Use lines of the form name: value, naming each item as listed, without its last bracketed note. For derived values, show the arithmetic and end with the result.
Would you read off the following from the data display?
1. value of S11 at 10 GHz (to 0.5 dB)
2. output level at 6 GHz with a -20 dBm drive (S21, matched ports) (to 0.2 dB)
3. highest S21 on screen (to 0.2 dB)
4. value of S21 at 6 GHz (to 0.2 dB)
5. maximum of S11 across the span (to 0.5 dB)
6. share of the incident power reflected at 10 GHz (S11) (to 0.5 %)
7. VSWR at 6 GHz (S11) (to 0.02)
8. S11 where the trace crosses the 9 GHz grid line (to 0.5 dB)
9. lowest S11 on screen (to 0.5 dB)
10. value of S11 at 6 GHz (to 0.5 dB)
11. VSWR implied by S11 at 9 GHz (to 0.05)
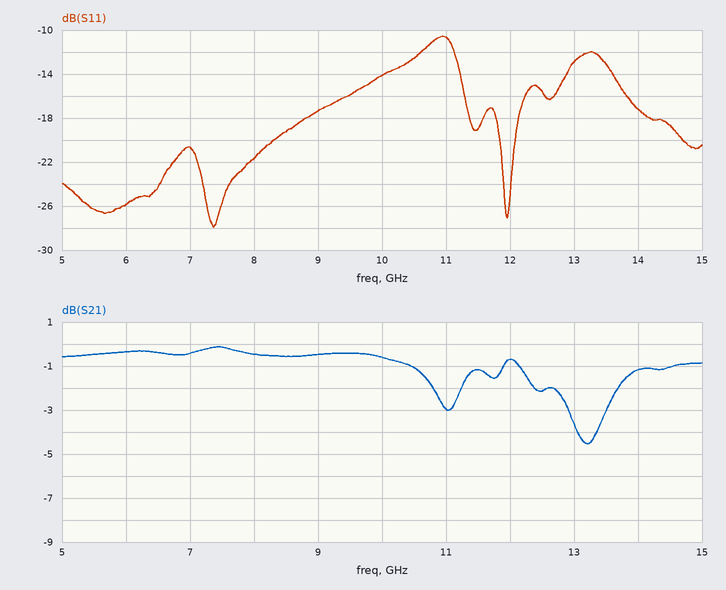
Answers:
value of S11 at 10 GHz: -14.0 dB
output level at 6 GHz with a -20 dBm drive (S21, matched ports): -20 dBm + (-0.4 dB) = -20.4 dBm
highest S21 on screen: -0.2 dB
value of S21 at 6 GHz: -0.4 dB
maximum of S11 across the span: -10.5 dB
share of the incident power reflected at 10 GHz (S11): 10^(-14/10) ≈ 4.0 %
VSWR at 6 GHz (S11): |Γ| = 10^(-26/20) = 0.0501; VSWR = (1 + 0.0501)/(1 − 0.0501) ≈ 1.11, so 1.10 to the nearest 0.02
S11 where the trace crosses the 9 GHz grid line: -17.5 dB
lowest S11 on screen: -28.0 dB
value of S11 at 6 GHz: -26.0 dB
VSWR implied by S11 at 9 GHz: |Γ| = 10^(-17.5/20) = 0.1334; VSWR = (1 + 0.1334)/(1 − 0.1334) ≈ 1.31, so 1.30 to the nearest 0.05
